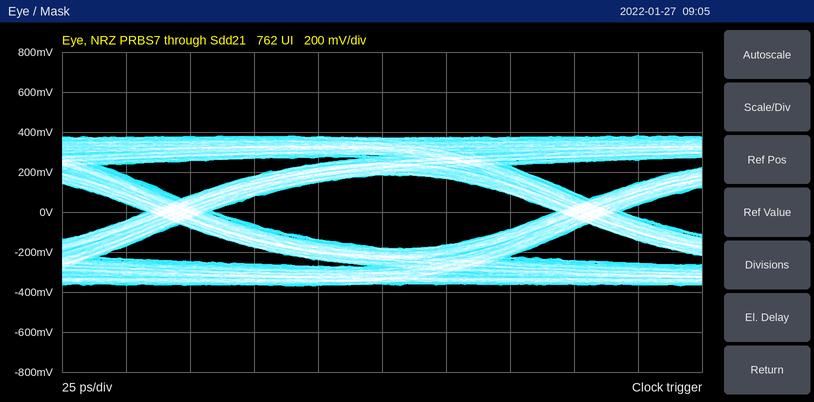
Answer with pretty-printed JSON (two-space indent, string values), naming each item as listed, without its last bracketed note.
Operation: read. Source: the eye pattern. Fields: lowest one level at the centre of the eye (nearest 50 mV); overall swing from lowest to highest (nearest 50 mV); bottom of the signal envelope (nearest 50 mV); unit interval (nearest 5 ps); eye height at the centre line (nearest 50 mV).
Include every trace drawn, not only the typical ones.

{
  "lowest one level at the centre of the eye": "200 mV",
  "overall swing from lowest to highest": "750 mV",
  "bottom of the signal envelope": "-350 mV",
  "unit interval": "160 ps",
  "eye height at the centre line": "350 mV"
}
